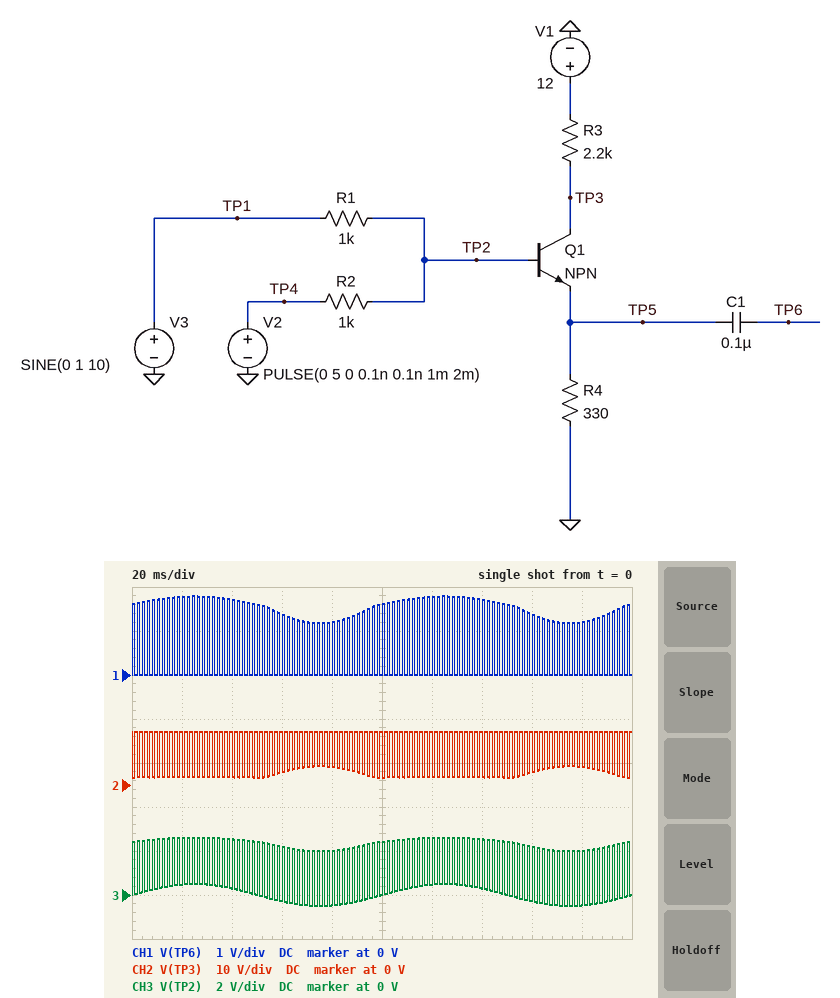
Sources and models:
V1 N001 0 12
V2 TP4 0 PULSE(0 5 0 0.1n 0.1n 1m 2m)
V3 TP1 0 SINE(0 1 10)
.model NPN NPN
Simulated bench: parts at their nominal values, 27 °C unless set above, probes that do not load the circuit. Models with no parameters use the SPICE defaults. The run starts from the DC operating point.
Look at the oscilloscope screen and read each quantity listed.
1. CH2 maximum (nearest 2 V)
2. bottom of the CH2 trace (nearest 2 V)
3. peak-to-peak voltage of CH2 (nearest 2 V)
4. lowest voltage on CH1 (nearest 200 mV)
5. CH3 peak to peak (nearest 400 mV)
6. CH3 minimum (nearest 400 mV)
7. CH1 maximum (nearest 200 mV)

12 V
2 V
10 V
0 V
3.2 V
-400 mV
1.8 V
